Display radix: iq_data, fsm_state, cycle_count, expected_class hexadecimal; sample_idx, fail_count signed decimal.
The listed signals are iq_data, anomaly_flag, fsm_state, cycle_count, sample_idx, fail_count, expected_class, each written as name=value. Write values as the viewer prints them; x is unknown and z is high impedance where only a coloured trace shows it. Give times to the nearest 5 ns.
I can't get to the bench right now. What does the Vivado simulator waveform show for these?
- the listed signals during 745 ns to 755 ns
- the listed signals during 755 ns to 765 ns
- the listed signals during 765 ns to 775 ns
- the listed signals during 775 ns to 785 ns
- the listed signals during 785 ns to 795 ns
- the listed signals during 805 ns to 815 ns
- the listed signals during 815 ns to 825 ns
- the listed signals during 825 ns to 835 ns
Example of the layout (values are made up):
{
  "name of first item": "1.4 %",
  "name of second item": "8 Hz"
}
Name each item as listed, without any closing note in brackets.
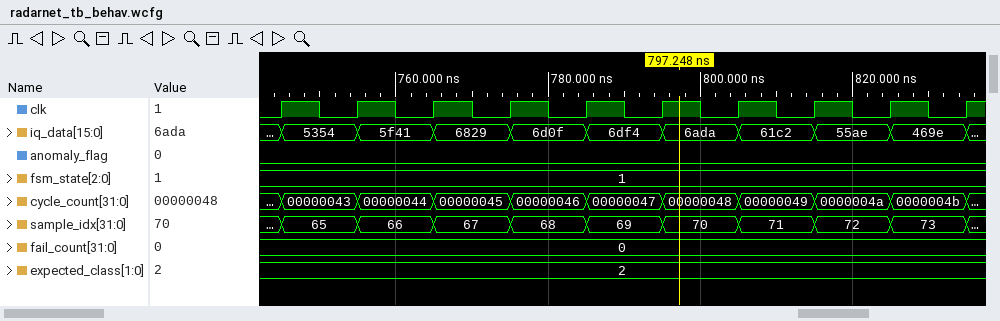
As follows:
{
  "the listed signals during 745 ns to 755 ns": "iq_data=5354, anomaly_flag=0, fsm_state=1, cycle_count=00000043, sample_idx=65, fail_count=0, expected_class=2",
  "the listed signals during 755 ns to 765 ns": "iq_data=5f41, anomaly_flag=0, fsm_state=1, cycle_count=00000044, sample_idx=66, fail_count=0, expected_class=2",
  "the listed signals during 765 ns to 775 ns": "iq_data=6829, anomaly_flag=0, fsm_state=1, cycle_count=00000045, sample_idx=67, fail_count=0, expected_class=2",
  "the listed signals during 775 ns to 785 ns": "iq_data=6d0f, anomaly_flag=0, fsm_state=1, cycle_count=00000046, sample_idx=68, fail_count=0, expected_class=2",
  "the listed signals during 785 ns to 795 ns": "iq_data=6df4, anomaly_flag=0, fsm_state=1, cycle_count=00000047, sample_idx=69, fail_count=0, expected_class=2",
  "the listed signals during 805 ns to 815 ns": "iq_data=61c2, anomaly_flag=0, fsm_state=1, cycle_count=00000049, sample_idx=71, fail_count=0, expected_class=2",
  "the listed signals during 815 ns to 825 ns": "iq_data=55ae, anomaly_flag=0, fsm_state=1, cycle_count=0000004a, sample_idx=72, fail_count=0, expected_class=2",
  "the listed signals during 825 ns to 835 ns": "iq_data=469e, anomaly_flag=0, fsm_state=1, cycle_count=0000004b, sample_idx=73, fail_count=0, expected_class=2"
}
